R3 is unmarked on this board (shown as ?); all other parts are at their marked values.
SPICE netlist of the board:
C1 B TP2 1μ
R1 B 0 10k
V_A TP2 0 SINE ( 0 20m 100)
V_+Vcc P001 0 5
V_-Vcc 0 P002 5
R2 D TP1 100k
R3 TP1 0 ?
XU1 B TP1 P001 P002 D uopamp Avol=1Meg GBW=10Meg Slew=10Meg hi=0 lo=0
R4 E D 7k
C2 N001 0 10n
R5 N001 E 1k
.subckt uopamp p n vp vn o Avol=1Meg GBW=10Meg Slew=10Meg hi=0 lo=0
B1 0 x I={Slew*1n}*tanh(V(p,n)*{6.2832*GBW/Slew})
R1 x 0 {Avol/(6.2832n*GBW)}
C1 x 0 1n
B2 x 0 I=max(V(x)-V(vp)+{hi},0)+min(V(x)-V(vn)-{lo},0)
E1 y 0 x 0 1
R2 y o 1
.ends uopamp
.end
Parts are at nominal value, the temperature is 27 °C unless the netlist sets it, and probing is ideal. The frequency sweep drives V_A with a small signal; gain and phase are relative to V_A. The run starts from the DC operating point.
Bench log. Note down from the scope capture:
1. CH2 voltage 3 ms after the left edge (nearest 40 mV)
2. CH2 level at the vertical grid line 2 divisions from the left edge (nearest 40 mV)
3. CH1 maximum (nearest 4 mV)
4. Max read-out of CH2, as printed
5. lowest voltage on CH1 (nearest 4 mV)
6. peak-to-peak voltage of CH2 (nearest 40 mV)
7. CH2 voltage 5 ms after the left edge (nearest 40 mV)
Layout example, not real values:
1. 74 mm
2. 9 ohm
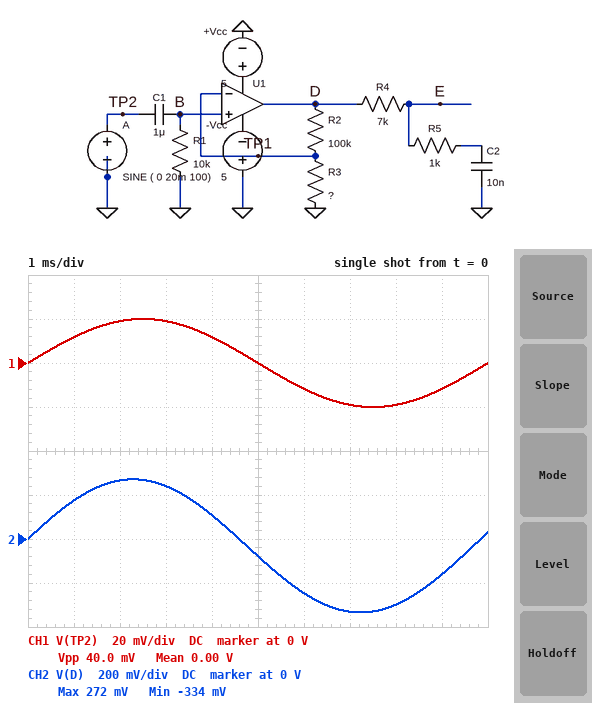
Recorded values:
1. 240 mV
2. 280 mV
3. 20 mV
4. 272 mV
5. -20 mV
6. 600 mV
7. -80 mV
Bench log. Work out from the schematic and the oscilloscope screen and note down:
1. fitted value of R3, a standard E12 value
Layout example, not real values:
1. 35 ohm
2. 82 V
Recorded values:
1. 6.8 kΩ
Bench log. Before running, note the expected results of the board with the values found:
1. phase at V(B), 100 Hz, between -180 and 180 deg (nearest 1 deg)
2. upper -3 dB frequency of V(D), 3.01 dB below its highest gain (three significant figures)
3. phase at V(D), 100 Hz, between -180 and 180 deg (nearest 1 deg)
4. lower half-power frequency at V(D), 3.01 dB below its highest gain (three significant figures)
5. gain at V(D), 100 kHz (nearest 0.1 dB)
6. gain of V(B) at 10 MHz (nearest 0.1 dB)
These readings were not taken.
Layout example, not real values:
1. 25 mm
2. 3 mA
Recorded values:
1. 9 deg
2. 637 kHz
3. 9 deg
4. 15.9 Hz
5. 23.8 dB
6. 0 dB
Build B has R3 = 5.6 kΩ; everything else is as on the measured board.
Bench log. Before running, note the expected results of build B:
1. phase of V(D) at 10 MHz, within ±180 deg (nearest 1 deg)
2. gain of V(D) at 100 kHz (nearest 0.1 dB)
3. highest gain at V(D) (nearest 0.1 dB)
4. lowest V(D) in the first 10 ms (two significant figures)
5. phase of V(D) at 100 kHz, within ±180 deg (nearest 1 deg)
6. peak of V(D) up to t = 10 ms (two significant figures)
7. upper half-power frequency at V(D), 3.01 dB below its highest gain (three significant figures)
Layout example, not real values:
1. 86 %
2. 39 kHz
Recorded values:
1. -87 deg
2. 25.4 dB
3. 25.5 dB
4. -400 mV
5. -11 deg
6. 330 mV
7. 530 kHz
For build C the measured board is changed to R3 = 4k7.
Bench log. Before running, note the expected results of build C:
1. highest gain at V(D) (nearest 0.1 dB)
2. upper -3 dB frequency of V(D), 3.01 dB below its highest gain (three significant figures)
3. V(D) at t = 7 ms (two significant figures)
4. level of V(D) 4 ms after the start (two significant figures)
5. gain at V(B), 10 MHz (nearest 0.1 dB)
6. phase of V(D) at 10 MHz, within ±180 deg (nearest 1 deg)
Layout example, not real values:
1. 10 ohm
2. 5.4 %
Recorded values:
1. 27.0 dB
2. 449 kHz
3. -470 mV
4. 150 mV
5. 0 dB
6. -87 deg
